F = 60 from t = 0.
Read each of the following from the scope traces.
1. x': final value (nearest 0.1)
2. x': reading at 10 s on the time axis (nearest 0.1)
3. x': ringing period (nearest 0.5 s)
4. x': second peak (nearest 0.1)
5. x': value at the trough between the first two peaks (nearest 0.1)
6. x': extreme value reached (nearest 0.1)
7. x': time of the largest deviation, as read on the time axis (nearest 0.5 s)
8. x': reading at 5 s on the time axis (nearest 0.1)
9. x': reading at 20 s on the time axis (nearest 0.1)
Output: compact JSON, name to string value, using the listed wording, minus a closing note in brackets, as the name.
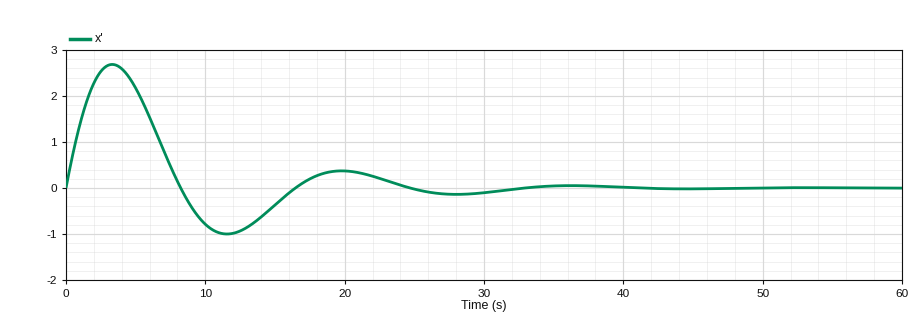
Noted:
{"x': final value": "0.0", "x': reading at 10 s on the time axis": "-0.8", "x': ringing period": "16.5 s", "x': second peak": "0.4", "x': value at the trough between the first two peaks": "-1.0", "x': extreme value reached": "2.7", "x': time of the largest deviation, as read on the time axis": "3.5 s", "x': reading at 5 s on the time axis": "2.2", "x': reading at 20 s on the time axis": "0.4"}
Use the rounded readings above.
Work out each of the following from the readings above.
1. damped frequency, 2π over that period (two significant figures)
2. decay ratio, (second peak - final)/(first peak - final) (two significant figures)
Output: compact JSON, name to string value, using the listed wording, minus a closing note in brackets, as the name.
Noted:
{"damped frequency, 2π over that period": "0.38 rad/s", "decay ratio, (second peak - final)/(first peak - final)": "0.15"}
